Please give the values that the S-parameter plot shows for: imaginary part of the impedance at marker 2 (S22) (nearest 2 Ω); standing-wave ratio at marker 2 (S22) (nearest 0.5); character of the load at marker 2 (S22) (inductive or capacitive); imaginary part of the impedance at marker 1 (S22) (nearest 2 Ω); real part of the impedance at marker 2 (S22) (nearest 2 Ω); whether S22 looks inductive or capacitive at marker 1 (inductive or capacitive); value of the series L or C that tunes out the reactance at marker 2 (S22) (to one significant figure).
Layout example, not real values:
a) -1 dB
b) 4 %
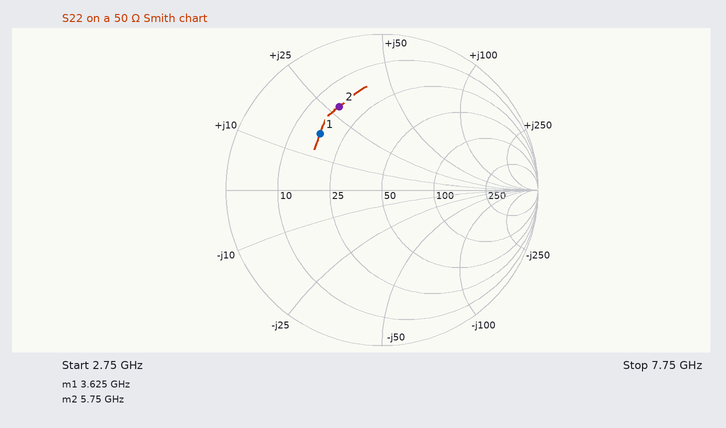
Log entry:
a) +28 Ω
b) 4.0
c) inductive
d) +18 Ω
e) 16 Ω
f) inductive
g) 1.0 pF
